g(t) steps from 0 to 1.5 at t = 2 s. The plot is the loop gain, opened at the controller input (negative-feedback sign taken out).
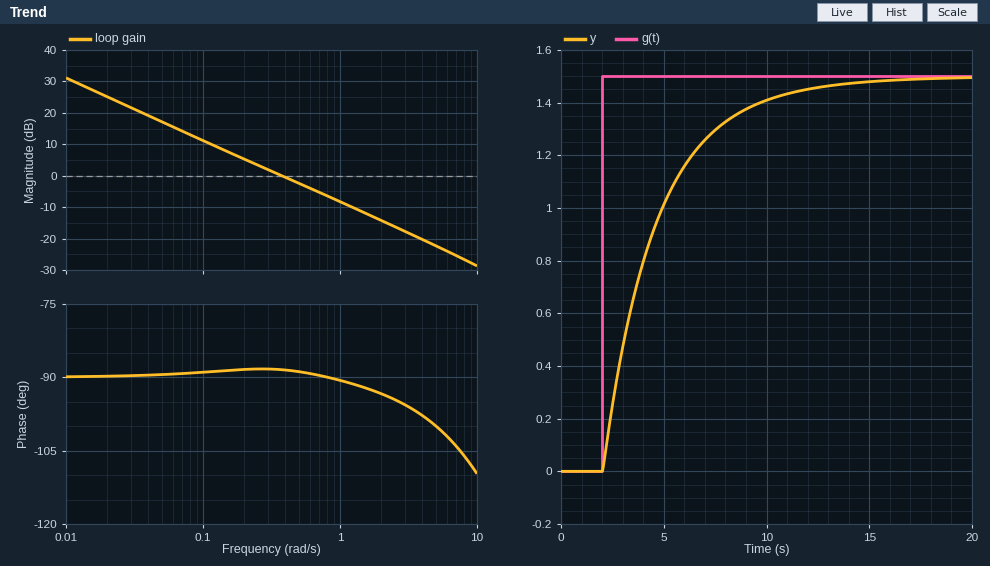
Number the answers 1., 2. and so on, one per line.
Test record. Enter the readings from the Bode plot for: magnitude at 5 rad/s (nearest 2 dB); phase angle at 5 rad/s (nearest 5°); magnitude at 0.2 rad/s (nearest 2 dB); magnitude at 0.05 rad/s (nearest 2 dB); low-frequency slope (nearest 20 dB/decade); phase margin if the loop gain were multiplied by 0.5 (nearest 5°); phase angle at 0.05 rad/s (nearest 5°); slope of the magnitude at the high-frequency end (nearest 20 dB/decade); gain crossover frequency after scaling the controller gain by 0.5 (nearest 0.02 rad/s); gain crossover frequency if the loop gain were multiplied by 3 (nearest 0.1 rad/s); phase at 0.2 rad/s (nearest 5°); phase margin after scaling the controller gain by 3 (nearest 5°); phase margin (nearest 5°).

1. -22 dB
2. -100°
3. 6 dB
4. 18 dB
5. -20 dB/decade
6. 90°
7. -90°
8. -20 dB/decade
9. 0.18 rad/s
10. 1.2 rad/s
11. -90°
12. 90°
13. 90°
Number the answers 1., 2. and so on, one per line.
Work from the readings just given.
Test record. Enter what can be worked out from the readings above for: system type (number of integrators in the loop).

1. 1
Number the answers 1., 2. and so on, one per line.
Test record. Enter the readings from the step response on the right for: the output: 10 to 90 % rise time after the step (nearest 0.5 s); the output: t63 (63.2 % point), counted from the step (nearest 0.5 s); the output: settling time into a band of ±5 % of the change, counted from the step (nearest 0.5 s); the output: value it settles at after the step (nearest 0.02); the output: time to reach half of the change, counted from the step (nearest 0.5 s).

1. 6.0 s
2. 2.5 s
3. 8.5 s
4. 1.50
5. 2.0 s
